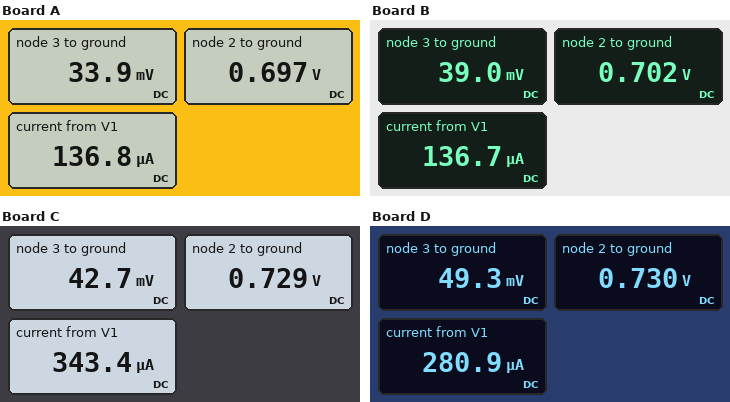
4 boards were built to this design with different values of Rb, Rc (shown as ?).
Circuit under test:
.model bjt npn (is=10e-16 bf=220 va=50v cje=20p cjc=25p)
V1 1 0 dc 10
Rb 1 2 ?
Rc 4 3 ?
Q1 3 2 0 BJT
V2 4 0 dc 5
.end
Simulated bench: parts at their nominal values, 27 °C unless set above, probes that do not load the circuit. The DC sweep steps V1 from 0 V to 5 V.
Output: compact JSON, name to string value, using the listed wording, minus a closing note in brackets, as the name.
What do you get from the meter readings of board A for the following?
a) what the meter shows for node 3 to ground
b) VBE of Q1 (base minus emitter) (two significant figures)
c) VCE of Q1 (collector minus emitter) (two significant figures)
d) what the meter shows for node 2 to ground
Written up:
{"what the meter shows for node 3 to ground": "33.9 mV", "VBE of Q1 (base minus emitter)": "700 mV", "VCE of Q1 (collector minus emitter)": "34 mV", "what the meter shows for node 2 to ground": "0.697 V"}
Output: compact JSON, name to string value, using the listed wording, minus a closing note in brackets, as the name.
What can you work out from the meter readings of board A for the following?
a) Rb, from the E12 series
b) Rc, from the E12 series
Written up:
{"Rb, from the E12 series": "68 kΩ", "Rc, from the E12 series": "22 kΩ"}
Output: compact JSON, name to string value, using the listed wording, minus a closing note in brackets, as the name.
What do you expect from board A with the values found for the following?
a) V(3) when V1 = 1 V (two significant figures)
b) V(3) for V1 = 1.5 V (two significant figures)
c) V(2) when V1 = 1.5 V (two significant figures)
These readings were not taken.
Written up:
{"V(3) when V1 = 1 V": "110 mV", "V(3) for V1 = 1.5 V": "81 mV", "V(2) when V1 = 1.5 V": "680 mV"}
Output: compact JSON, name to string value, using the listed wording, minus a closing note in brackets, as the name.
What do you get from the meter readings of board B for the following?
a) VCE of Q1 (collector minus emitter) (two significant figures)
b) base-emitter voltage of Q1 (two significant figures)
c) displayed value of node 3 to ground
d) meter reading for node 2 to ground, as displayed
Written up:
{"VCE of Q1 (collector minus emitter)": "39 mV", "base-emitter voltage of Q1": "700 mV", "displayed value of node 3 to ground": "39.0 mV", "meter reading for node 2 to ground, as displayed": "0.702 V"}
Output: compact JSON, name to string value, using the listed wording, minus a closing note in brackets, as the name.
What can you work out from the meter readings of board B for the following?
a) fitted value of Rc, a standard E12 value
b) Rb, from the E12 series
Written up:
{"fitted value of Rc, a standard E12 value": "15 kΩ", "Rb, from the E12 series": "68 kΩ"}
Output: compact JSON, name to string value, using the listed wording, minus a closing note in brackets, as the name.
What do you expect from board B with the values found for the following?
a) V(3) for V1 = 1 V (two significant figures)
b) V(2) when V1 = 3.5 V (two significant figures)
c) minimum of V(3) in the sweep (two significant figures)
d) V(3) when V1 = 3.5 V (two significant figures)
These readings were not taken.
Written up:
{"V(3) for V1 = 1 V": "120 mV", "V(2) when V1 = 3.5 V": "690 mV", "minimum of V(3) in the sweep": "52 mV", "V(3) when V1 = 3.5 V": "61 mV"}
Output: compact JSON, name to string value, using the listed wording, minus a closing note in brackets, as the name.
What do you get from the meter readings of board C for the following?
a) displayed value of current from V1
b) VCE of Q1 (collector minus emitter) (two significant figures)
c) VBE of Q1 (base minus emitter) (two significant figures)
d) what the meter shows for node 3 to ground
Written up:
{"displayed value of current from V1": "343.4 µA", "VCE of Q1 (collector minus emitter)": "43 mV", "VBE of Q1 (base minus emitter)": "730 mV", "what the meter shows for node 3 to ground": "42.7 mV"}
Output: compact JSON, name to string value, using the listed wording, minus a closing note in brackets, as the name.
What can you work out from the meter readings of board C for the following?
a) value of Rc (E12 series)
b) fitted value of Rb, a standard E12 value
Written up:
{"value of Rc": "4.7 kΩ", "fitted value of Rb, a standard E12 value": "27 kΩ"}
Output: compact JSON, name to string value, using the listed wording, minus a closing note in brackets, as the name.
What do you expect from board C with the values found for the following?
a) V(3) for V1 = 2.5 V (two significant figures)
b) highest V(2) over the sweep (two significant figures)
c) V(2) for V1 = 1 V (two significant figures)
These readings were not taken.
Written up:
{"V(3) for V1 = 2.5 V": "77 mV", "highest V(2) over the sweep": "720 mV", "V(2) for V1 = 1 V": "720 mV"}
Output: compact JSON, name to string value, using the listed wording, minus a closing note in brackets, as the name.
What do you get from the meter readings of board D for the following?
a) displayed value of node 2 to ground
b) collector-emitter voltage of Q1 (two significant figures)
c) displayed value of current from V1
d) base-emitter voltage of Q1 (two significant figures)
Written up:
{"displayed value of node 2 to ground": "0.730 V", "collector-emitter voltage of Q1": "49 mV", "displayed value of current from V1": "280.9 µA", "base-emitter voltage of Q1": "730 mV"}
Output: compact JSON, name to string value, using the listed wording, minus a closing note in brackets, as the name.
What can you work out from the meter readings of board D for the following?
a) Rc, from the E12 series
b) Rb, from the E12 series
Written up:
{"Rc, from the E12 series": "3.9 kΩ", "Rb, from the E12 series": "33 kΩ"}
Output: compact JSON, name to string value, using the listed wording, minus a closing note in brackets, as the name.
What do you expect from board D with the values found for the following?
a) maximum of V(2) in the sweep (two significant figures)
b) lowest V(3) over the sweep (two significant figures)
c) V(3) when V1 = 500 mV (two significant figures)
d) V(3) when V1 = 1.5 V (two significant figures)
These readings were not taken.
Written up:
{"maximum of V(2) in the sweep": "730 mV", "lowest V(3) over the sweep": "65 mV", "V(3) when V1 = 500 mV": "5.0 V", "V(3) when V1 = 1.5 V": "110 mV"}
